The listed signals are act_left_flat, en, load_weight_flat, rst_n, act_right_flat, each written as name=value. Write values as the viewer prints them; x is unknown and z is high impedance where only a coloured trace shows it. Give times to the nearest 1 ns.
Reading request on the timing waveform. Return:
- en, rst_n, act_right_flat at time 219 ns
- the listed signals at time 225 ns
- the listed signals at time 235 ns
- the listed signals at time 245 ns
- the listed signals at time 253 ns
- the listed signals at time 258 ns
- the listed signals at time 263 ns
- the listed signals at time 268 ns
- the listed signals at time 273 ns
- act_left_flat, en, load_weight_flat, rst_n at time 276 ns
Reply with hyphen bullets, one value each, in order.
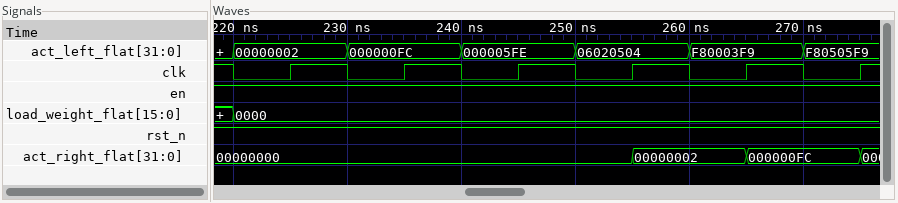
- en=1, rst_n=1, act_right_flat=00000000
- act_left_flat=00000002, en=1, load_weight_flat=0000, rst_n=1, act_right_flat=00000000
- act_left_flat=000000FC, en=1, load_weight_flat=0000, rst_n=1, act_right_flat=00000000
- act_left_flat=000005FE, en=1, load_weight_flat=0000, rst_n=1, act_right_flat=00000000
- act_left_flat=06020504, en=1, load_weight_flat=0000, rst_n=1, act_right_flat=00000000
- act_left_flat=06020504, en=1, load_weight_flat=0000, rst_n=1, act_right_flat=00000002
- act_left_flat=F80003F9, en=1, load_weight_flat=0000, rst_n=1, act_right_flat=00000002
- act_left_flat=F80003F9, en=1, load_weight_flat=0000, rst_n=1, act_right_flat=000000FC
- act_left_flat=F80505F9, en=1, load_weight_flat=0000, rst_n=1, act_right_flat=000000FC
- act_left_flat=F80505F9, en=1, load_weight_flat=0000, rst_n=1
